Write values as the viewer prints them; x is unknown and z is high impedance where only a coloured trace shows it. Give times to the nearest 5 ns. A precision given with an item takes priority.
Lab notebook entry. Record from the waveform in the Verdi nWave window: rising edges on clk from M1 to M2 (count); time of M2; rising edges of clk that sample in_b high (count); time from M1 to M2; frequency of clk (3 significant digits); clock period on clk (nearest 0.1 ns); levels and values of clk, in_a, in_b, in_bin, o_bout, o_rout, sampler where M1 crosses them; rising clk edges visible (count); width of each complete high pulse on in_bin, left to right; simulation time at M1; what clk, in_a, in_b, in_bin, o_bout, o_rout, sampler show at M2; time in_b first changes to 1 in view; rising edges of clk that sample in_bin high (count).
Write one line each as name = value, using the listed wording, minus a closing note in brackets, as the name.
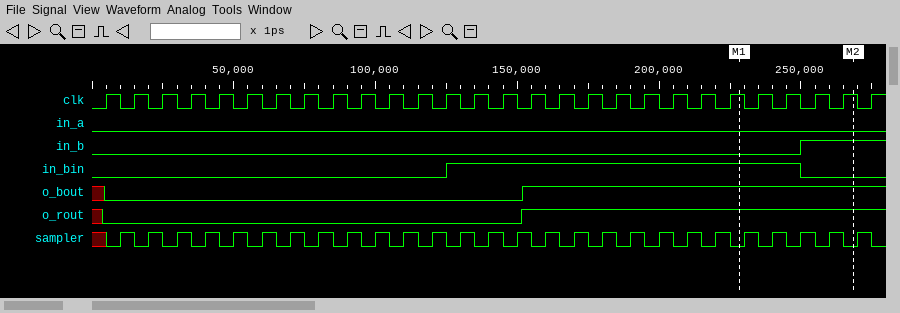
rising edges on clk from M1 to M2 = 4
time of M2 = 270 ns
rising edges of clk that sample in_b high = 3
time from M1 to M2 = 40 ns
frequency of clk = 100 MHz
clock period on clk = 10 ns
levels and values of clk, in_a, in_b, in_bin, o_bout, o_rout, sampler where M1 crosses them = clk=1, in_a=0, in_b=0, in_bin=1, o_bout=1, o_rout=1, sampler=0
rising clk edges visible = 28
width of each complete high pulse on in_bin, left to right = 125 ns
simulation time at M1 = 230 ns
what clk, in_a, in_b, in_bin, o_bout, o_rout, sampler show at M2 = clk=1, in_a=0, in_b=1, in_bin=0, o_bout=1, o_rout=1, sampler=0
time in_b first changes to 1 in view = 250 ns
rising edges of clk that sample in_bin high = 12
